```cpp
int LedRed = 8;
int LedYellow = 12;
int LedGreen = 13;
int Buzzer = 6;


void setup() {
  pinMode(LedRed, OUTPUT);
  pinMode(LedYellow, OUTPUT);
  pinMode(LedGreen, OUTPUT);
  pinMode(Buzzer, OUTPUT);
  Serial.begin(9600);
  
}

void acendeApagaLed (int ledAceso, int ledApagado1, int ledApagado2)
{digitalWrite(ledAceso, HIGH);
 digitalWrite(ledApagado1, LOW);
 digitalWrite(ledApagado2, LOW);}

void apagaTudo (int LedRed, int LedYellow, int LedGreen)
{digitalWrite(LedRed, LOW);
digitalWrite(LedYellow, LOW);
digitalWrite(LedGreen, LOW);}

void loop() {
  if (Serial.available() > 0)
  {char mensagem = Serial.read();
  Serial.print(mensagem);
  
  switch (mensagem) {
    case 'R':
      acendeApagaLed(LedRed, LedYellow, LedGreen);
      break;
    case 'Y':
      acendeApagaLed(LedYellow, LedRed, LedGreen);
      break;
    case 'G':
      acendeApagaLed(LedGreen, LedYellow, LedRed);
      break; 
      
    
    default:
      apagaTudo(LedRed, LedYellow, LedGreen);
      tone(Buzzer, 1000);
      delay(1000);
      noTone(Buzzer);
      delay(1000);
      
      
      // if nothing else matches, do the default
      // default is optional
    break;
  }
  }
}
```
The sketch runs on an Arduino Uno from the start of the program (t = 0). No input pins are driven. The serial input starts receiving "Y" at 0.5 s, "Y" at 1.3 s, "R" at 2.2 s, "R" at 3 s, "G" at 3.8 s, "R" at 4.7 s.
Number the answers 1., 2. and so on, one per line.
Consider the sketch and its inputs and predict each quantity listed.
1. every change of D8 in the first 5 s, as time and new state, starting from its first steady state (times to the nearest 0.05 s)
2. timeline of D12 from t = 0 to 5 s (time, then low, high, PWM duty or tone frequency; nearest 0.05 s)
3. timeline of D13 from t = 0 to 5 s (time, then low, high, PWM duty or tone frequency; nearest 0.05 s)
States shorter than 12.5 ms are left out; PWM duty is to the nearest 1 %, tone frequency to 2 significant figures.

1. 0 s low; 2.2 s high; 3.8 s low; 4.7 s high
2. 0 s low; 0.5 s high; 2.2 s low
3. 0 s low; 3.8 s high; 4.7 s low
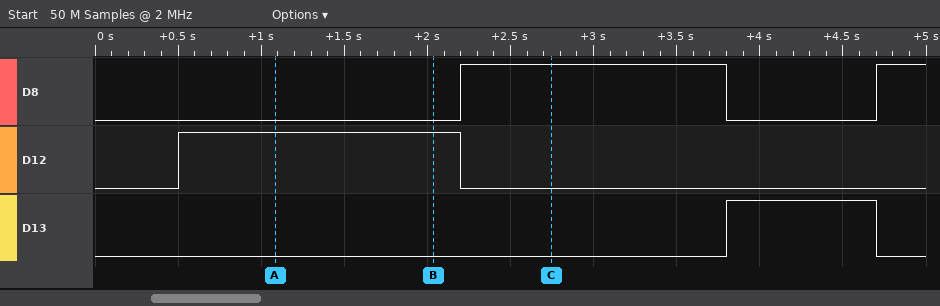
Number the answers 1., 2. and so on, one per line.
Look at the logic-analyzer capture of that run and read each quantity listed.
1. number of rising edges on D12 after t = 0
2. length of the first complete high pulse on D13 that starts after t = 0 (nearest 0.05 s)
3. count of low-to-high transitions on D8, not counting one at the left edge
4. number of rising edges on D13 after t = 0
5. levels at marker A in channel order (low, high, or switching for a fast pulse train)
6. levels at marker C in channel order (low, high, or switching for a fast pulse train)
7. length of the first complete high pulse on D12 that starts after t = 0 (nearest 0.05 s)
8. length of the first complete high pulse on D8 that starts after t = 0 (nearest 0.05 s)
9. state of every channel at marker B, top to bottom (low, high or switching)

1. 1
2. 0.90 s
3. 2
4. 1
5. D8 low, D12 high, D13 low
6. D8 high, D12 low, D13 low
7. 1.70 s
8. 1.60 s
9. D8 low, D12 high, D13 low
